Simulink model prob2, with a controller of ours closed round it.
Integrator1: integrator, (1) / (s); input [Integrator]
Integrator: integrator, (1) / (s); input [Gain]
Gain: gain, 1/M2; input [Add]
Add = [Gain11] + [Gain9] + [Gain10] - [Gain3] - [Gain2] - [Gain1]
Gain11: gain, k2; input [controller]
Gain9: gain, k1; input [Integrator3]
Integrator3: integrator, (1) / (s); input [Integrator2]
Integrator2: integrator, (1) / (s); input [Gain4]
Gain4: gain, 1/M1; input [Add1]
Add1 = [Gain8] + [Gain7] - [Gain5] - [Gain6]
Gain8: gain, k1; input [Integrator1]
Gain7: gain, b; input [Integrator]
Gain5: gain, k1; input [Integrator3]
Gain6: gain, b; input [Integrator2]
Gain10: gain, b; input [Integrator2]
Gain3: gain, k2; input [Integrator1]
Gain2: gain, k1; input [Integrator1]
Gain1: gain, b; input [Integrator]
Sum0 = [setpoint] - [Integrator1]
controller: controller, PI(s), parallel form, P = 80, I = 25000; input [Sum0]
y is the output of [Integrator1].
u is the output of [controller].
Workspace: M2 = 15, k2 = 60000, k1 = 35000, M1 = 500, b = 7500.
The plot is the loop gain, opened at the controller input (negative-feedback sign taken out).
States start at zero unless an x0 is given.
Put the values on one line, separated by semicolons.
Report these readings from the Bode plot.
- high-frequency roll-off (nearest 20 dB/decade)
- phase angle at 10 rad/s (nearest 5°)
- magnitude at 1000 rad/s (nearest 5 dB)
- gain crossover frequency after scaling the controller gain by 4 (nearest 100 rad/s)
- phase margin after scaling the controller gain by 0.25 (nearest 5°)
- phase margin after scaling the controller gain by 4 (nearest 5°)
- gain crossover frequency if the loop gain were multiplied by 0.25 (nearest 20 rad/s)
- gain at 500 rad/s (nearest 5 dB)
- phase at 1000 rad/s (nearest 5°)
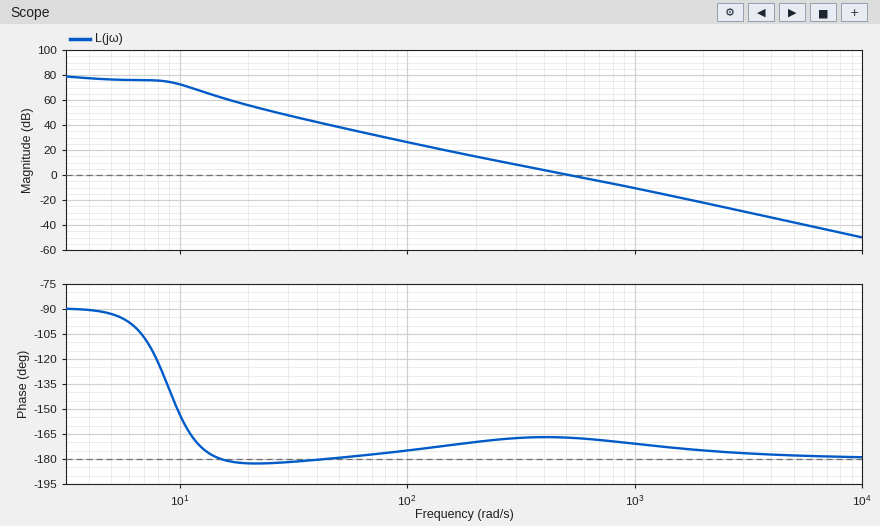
-40 dB/decade; -155°; -10 dB; 1100 rad/s; 10°; 10°; 240 rad/s; 0 dB; -170°
